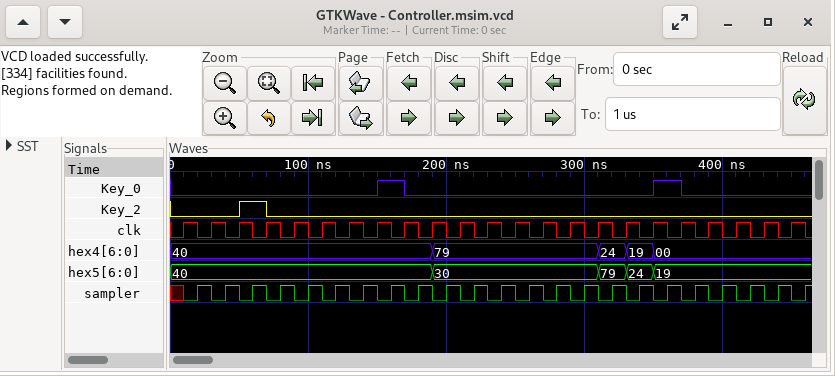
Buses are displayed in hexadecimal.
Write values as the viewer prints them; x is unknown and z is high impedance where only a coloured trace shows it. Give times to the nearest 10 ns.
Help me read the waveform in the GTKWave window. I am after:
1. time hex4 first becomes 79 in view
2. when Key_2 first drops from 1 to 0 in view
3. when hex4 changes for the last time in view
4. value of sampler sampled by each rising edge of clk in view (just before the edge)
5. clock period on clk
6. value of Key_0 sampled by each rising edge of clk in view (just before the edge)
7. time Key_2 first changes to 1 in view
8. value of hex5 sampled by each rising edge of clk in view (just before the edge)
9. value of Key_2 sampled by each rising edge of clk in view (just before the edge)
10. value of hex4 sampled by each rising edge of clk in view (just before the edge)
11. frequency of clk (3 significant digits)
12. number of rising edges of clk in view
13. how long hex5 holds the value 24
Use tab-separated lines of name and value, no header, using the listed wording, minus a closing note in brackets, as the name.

time hex4 first becomes 79 in view	190 ns
when Key_2 first drops from 1 to 0 in view	70 ns
when hex4 changes for the last time in view	350 ns
value of sampler sampled by each rising edge of clk in view	x 1 1 1 1 1 1 1 1 1 1 1 1 1 1 1 1 1 1 1 1 1 1
clock period on clk	20 ns
value of Key_0 sampled by each rising edge of clk in view	0 0 0 0 0 0 0 0 1 0 0 0 0 0 0 0 0 0 1 0 0 0 0
time Key_2 first changes to 1 in view	50 ns
value of hex5 sampled by each rising edge of clk in view	40, 40, 40, 40, 40, 40, 40, 40, 40, 40, 30, 30, 30, 30, 30, 30, 79, 24, 19, 19, 19, 19, 19
value of Key_2 sampled by each rising edge of clk in view	0 0 0 1 0 0 0 0 0 0 0 0 0 0 0 0 0 0 0 0 0 0 0
value of hex4 sampled by each rising edge of clk in view	40, 40, 40, 40, 40, 40, 40, 40, 40, 40, 79, 79, 79, 79, 79, 79, 24, 19, 00, 00, 00, 00, 00
frequency of clk	50.0 MHz
number of rising edges of clk in view	23
how long hex5 holds the value 24	20 ns
